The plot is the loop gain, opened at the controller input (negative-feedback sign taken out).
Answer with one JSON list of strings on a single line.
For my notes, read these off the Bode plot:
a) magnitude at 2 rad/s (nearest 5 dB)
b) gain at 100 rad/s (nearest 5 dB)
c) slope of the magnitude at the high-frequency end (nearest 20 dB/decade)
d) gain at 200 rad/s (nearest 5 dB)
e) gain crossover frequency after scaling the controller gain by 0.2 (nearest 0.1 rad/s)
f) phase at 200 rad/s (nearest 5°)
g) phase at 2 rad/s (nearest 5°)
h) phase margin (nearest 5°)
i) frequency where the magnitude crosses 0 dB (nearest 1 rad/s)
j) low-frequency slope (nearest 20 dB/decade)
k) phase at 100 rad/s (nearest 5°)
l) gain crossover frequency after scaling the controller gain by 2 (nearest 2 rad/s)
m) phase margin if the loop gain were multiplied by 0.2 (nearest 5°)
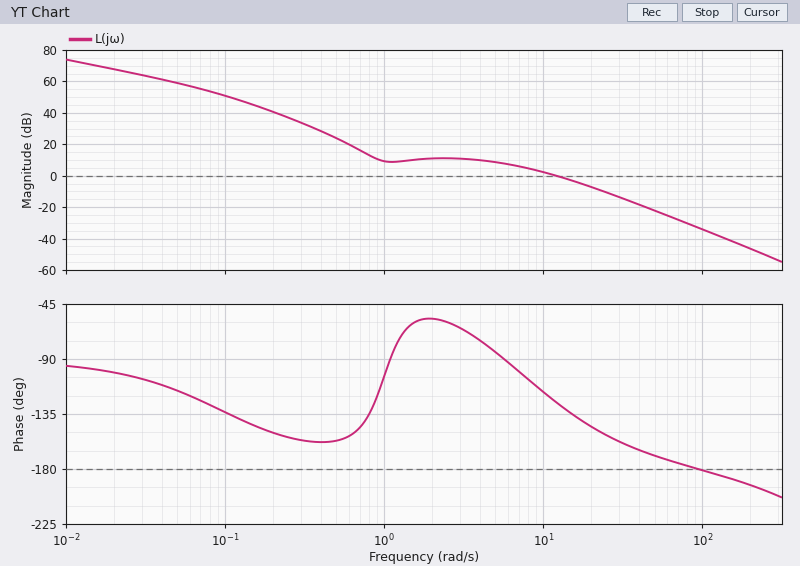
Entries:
["10 dB", "-35 dB", "-40 dB/decade", "-45 dB", "0.8 rad/s", "-195°", "-55°", "55°", "12 rad/s", "-20 dB/decade", "-180°", "18 rad/s", "40°"]
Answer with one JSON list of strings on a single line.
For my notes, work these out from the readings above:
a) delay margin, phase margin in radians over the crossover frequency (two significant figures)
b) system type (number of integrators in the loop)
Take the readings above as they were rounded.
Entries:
["0.080 s", "1"]
